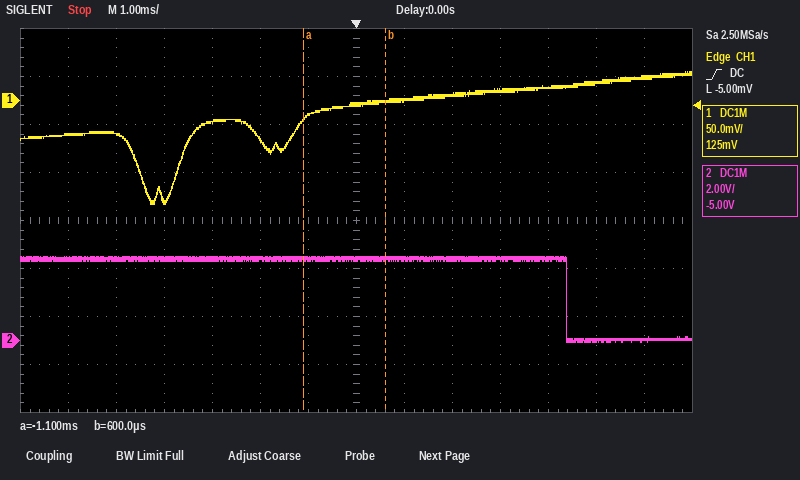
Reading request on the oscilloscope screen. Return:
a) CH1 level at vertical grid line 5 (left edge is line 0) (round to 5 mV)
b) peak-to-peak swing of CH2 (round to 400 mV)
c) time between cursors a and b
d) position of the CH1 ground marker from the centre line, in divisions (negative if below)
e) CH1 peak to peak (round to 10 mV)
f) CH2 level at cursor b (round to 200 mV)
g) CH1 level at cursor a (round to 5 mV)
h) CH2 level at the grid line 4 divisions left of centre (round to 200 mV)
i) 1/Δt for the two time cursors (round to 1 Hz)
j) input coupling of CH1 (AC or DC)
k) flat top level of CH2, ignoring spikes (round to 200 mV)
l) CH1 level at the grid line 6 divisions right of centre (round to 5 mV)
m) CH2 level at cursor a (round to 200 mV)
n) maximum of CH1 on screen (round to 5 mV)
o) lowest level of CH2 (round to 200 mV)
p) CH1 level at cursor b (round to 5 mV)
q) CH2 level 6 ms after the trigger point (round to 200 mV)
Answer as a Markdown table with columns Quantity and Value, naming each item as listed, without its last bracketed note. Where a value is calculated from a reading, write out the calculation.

| Quantity | Value |
|---|---|
| CH1 level at vertical grid line 5 (left edge is line 0) | -40 mV |
| peak-to-peak swing of CH2 | 3.6 V |
| time between cursors a and b | 600 µs − (-1.1 ms) = 1.7 ms |
| position of the CH1 ground marker from the centre line, in divisions | +2.5 div |
| CH1 peak to peak | 140 mV |
| CH2 level at cursor b | 3.4 V |
| CH1 level at cursor a | -20 mV |
| CH2 level at the grid line 4 divisions left of centre | 3.4 V |
| 1/Δt for the two time cursors | 1 / 1.7 ms ≈ 588 Hz |
| input coupling of CH1 | DC |
| flat top level of CH2, ignoring spikes | 3.4 V |
| CH1 level at the grid line 6 divisions right of centre | 25 mV |
| CH2 level at cursor a | 3.4 V |
| maximum of CH1 on screen | 30 mV |
| lowest level of CH2 | 0.0 V |
| CH1 level at cursor b | 0 mV |
| CH2 level 6 ms after the trigger point | 0.0 V |
